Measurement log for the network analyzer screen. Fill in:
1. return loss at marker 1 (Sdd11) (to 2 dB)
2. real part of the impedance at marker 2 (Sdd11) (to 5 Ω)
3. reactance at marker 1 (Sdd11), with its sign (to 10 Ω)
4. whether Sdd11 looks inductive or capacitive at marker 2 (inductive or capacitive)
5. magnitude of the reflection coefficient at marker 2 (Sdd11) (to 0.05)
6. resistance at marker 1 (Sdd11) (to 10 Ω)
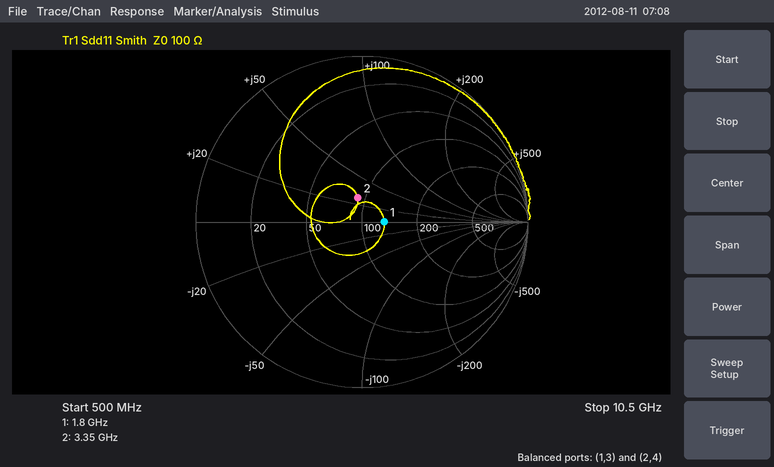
18 dB
90 Ω
0 Ω
inductive
0.15
130 Ω
